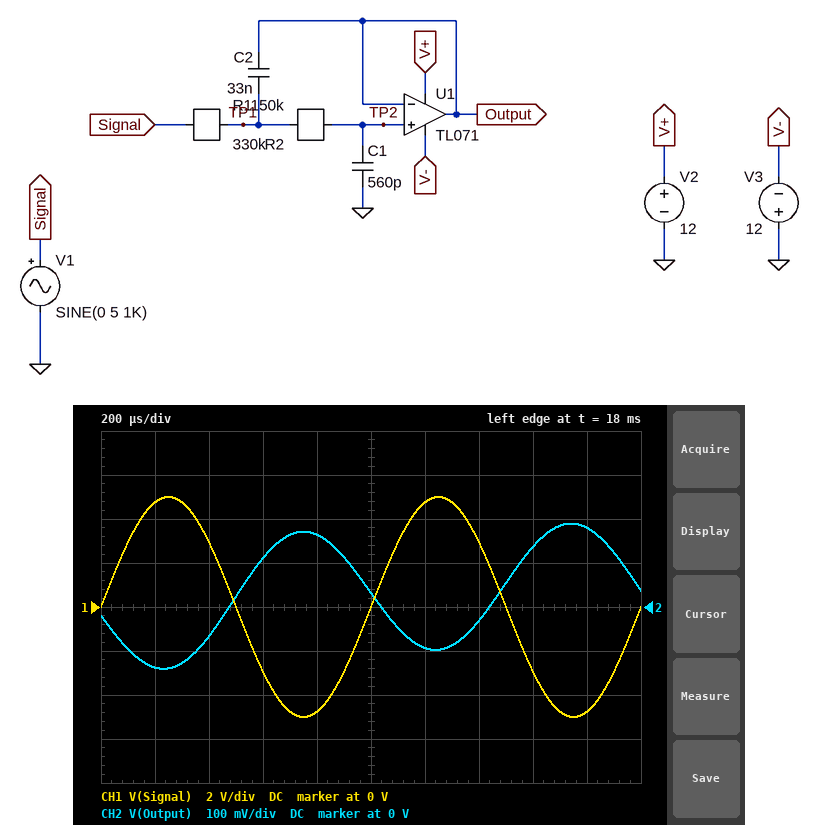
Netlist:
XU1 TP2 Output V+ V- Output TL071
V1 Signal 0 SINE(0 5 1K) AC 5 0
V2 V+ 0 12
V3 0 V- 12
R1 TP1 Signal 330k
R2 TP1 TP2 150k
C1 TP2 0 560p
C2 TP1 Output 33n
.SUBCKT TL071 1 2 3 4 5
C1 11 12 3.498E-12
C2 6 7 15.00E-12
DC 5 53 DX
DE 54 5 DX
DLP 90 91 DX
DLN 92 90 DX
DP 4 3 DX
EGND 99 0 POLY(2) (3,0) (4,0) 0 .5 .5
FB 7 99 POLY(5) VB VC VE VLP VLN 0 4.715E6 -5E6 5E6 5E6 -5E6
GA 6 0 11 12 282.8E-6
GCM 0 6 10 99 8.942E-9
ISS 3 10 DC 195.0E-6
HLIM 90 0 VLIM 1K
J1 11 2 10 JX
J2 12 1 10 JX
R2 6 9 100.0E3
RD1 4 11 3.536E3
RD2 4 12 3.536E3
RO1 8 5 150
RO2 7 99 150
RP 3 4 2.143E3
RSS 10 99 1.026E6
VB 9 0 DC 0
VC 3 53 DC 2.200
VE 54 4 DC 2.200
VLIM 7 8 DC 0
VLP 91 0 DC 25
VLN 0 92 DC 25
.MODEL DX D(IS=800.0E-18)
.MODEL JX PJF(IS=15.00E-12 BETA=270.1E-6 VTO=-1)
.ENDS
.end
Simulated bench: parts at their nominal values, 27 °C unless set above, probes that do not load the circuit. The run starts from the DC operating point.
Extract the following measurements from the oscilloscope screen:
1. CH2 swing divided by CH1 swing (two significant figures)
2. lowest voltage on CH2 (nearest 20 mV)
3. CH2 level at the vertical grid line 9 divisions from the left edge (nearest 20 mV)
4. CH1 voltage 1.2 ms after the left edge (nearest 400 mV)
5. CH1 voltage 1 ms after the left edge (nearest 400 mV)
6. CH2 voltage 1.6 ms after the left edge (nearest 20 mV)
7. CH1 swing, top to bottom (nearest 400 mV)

0.033
-140 mV
180 mV
4.8 V
0 V
140 mV
10.0 V
